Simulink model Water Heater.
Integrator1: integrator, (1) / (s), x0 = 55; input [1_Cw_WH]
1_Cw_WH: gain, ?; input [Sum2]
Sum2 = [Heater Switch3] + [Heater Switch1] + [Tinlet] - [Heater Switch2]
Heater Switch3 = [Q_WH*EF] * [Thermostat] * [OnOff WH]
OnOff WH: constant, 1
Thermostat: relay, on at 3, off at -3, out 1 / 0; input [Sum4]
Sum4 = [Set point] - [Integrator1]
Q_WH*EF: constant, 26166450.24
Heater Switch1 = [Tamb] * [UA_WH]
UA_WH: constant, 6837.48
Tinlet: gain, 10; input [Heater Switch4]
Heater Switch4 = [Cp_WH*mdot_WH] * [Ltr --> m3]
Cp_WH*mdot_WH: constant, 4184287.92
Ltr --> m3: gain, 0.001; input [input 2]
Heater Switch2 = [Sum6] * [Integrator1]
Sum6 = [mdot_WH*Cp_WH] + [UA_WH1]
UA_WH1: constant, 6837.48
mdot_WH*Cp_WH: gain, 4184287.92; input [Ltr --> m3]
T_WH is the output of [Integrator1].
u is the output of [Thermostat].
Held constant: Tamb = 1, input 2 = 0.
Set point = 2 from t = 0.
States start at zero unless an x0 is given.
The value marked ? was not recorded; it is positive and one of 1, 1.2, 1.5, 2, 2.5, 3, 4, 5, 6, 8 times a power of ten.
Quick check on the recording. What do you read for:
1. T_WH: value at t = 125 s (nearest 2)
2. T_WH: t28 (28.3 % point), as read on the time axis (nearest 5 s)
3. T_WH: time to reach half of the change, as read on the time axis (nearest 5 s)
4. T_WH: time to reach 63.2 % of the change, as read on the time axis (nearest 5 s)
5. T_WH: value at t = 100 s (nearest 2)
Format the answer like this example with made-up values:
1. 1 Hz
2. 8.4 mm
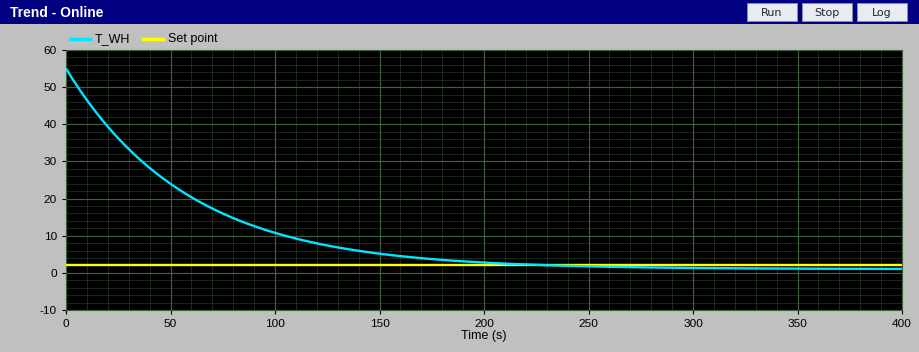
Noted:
1. 8
2. 20 s
3. 40 s
4. 60 s
5. 10
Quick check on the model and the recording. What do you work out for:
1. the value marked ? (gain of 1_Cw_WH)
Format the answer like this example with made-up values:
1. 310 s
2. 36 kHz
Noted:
1. 2.5e-06
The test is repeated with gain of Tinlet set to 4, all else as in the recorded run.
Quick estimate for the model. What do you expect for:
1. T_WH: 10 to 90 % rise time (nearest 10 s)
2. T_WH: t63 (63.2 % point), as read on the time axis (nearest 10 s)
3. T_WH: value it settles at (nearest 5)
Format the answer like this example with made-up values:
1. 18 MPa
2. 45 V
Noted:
1. 130 s
2. 60 s
3. 0
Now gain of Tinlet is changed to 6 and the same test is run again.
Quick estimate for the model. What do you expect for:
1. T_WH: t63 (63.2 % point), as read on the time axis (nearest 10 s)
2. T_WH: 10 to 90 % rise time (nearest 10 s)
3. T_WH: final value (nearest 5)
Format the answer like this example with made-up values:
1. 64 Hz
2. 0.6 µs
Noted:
1. 60 s
2. 130 s
3. 0
